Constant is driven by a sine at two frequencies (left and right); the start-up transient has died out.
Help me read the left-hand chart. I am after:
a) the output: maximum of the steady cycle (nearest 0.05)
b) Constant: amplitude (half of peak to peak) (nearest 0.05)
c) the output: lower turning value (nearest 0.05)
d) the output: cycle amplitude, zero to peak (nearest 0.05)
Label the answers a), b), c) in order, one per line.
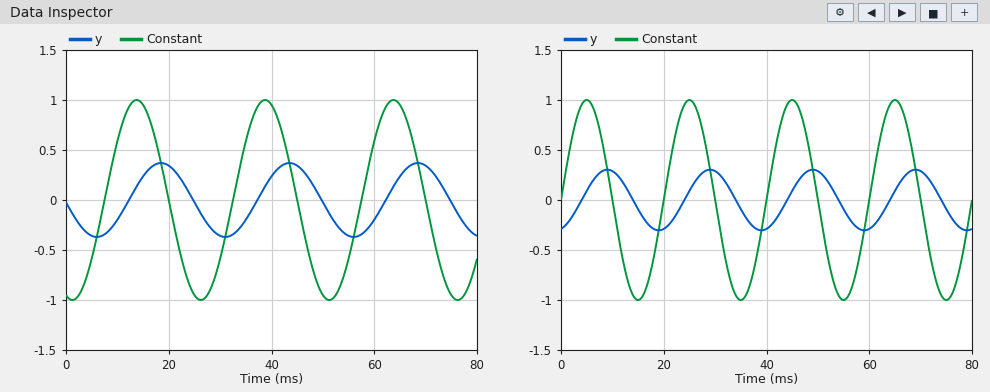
a) 0.35
b) 1.00
c) -0.35
d) 0.35
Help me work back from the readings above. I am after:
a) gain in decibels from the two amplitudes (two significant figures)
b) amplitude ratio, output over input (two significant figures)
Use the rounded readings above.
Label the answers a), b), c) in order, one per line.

a) -9.1 dB
b) 0.35
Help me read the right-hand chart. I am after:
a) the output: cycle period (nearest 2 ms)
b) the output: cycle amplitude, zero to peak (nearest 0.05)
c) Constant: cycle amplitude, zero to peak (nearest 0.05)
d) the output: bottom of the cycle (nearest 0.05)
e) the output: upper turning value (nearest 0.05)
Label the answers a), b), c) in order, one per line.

a) 20 ms
b) 0.30
c) 1.00
d) -0.30
e) 0.30
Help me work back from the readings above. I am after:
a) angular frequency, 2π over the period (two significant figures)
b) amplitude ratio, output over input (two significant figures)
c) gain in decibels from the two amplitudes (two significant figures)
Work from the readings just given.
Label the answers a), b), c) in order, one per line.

a) 0.31 rad/ms
b) 0.30
c) -10 dB
